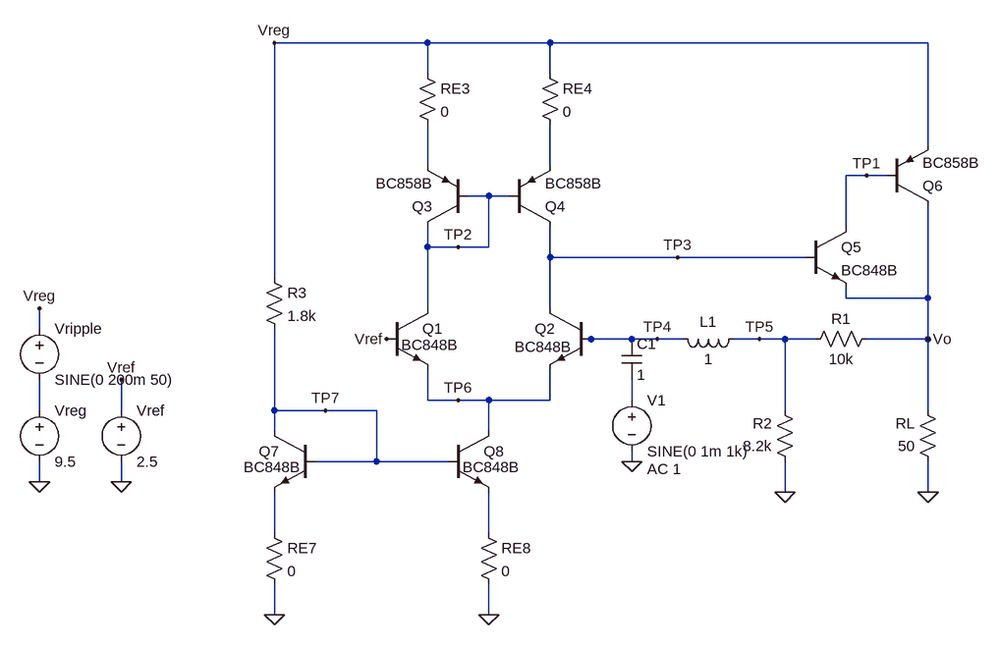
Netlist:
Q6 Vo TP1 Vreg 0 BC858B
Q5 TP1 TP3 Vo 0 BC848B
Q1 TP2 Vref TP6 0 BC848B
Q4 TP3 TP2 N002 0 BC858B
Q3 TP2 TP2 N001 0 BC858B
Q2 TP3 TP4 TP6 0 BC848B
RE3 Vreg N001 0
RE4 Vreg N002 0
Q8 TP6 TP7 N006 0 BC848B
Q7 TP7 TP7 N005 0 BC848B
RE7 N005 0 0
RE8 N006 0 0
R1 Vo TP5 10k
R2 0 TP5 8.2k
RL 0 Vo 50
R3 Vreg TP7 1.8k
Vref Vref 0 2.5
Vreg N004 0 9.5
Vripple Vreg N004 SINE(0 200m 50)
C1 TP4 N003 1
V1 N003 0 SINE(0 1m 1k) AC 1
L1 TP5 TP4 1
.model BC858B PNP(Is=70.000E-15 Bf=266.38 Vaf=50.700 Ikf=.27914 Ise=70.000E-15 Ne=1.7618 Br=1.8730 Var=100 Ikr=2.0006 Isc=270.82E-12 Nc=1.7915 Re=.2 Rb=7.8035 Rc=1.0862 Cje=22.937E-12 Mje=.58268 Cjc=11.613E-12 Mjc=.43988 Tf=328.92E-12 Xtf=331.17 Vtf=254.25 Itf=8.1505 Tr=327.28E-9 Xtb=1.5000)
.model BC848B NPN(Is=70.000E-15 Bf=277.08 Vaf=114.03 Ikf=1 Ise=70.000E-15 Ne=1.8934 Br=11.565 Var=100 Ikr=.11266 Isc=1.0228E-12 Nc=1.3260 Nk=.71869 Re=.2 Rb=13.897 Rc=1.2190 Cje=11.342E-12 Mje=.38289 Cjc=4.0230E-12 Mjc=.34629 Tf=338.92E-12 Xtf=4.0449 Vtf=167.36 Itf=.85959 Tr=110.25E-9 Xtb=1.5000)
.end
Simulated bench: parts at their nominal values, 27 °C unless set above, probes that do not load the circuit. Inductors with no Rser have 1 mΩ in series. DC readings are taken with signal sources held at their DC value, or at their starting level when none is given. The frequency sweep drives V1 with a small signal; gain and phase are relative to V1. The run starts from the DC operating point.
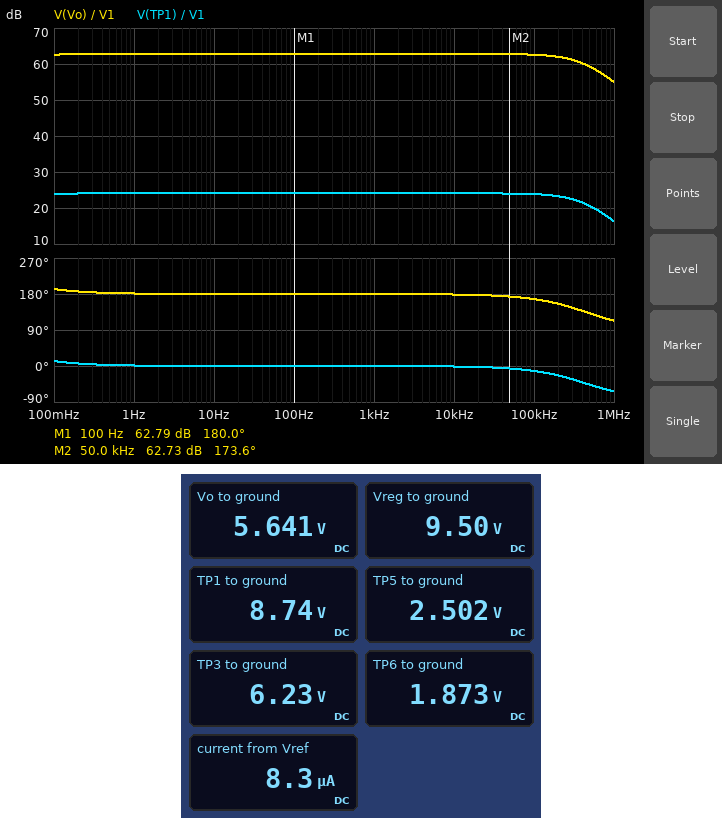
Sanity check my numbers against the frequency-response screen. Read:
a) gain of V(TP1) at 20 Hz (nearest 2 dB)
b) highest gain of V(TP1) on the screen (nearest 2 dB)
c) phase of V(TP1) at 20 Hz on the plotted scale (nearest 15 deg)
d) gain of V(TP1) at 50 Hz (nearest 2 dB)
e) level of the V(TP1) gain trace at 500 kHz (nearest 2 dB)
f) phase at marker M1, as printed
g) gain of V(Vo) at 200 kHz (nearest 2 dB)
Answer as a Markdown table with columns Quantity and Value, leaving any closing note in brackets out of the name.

| Quantity | Value |
|---|---|
| gain of V(TP1) at 20 Hz | 24 dB |
| highest gain of V(TP1) on the screen | 24 dB |
| phase of V(TP1) at 20 Hz on the plotted scale | 0 deg |
| gain of V(TP1) at 50 Hz | 24 dB |
| level of the V(TP1) gain trace at 500 kHz | 20 dB |
| phase at marker M1, as printed | 180.0 deg |
| gain of V(Vo) at 200 kHz | 62 dB |
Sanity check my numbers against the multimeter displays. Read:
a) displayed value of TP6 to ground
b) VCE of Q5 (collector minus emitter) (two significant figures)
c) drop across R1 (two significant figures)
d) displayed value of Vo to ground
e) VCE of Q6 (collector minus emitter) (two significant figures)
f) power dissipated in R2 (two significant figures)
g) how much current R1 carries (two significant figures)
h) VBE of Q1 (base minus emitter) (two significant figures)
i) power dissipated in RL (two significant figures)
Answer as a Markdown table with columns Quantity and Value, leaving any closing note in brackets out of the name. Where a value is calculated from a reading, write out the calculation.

| Quantity | Value |
|---|---|
| displayed value of TP6 to ground | 1.873 V |
| VCE of Q5 (collector minus emitter) | 8.74 V - 5.641 V = 3.1 V |
| drop across R1 | 5.641 V - 2.502 V = 3.1 V |
| displayed value of Vo to ground | 5.641 V |
| VCE of Q6 (collector minus emitter) | 5.641 V - 9.5 V = -3.9 V |
| power dissipated in R2 | (2.502 V)^2 / 8.2 kΩ = 760 µW |
| how much current R1 carries | (5.641 V - 2.502 V) / 10 kΩ = 310 µA |
| VBE of Q1 (base minus emitter) | 2.5 V - 1.873 V = 630 mV |
| power dissipated in RL | (5.641 V)^2 / 50 Ω = 640 mW |
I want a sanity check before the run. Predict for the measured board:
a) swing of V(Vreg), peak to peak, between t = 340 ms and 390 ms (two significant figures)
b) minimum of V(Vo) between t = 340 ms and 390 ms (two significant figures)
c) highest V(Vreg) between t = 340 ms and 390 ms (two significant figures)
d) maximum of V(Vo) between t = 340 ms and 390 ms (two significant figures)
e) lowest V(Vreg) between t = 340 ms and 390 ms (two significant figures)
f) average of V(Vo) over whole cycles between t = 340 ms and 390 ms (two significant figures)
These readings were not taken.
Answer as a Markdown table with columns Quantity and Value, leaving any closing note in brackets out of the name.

| Quantity | Value |
|---|---|
| swing of V(Vreg), peak to peak, between t = 340 ms and 390 ms | 400 mV |
| minimum of V(Vo) between t = 340 ms and 390 ms | 4.1 V |
| highest V(Vreg) between t = 340 ms and 390 ms | 9.7 V |
| maximum of V(Vo) between t = 340 ms and 390 ms | 7.2 V |
| lowest V(Vreg) between t = 340 ms and 390 ms | 9.3 V |
| average of V(Vo) over whole cycles between t = 340 ms and 390 ms | 5.7 V |
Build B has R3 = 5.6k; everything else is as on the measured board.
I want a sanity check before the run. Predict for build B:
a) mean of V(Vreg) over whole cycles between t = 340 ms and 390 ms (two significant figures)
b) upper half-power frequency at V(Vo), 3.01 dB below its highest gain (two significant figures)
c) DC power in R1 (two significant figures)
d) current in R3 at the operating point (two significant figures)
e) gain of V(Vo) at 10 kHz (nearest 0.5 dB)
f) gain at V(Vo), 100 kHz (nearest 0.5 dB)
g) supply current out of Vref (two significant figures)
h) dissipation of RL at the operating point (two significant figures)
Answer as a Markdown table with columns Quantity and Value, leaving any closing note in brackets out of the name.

| Quantity | Value |
|---|---|
| mean of V(Vreg) over whole cycles between t = 340 ms and 390 ms | 9.5 V |
| upper half-power frequency at V(Vo), 3.01 dB below its highest gain | 190 kHz |
| DC power in R1 | 950 µW |
| current in R3 at the operating point | 1.6 mA |
| gain of V(Vo) at 10 kHz | 62.5 dB |
| gain at V(Vo), 100 kHz | 61.5 dB |
| supply current out of Vref | 2.7 µA |
| dissipation of RL at the operating point | 620 mW |
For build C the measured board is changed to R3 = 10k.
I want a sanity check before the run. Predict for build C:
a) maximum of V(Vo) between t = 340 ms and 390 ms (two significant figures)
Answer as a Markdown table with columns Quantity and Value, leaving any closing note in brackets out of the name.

| Quantity | Value |
|---|---|
| maximum of V(Vo) between t = 340 ms and 390 ms | 7.1 V |
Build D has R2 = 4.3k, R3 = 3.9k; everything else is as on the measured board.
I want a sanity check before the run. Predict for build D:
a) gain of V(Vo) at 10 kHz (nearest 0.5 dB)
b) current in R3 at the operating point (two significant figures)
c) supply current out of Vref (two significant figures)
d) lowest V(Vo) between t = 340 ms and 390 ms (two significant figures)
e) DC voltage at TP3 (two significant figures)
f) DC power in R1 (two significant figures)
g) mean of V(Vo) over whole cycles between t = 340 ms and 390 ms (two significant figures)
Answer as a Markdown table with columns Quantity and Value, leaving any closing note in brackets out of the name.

| Quantity | Value |
|---|---|
| gain of V(Vo) at 10 kHz | 62.5 dB |
| current in R3 at the operating point | 2.3 mA |
| supply current out of Vref | 4.0 µA |
| lowest V(Vo) between t = 340 ms and 390 ms | 6.8 V |
| DC voltage at TP3 | 9.0 V |
| DC power in R1 | 3.4 mW |
| mean of V(Vo) over whole cycles between t = 340 ms and 390 ms | 8.1 V |
